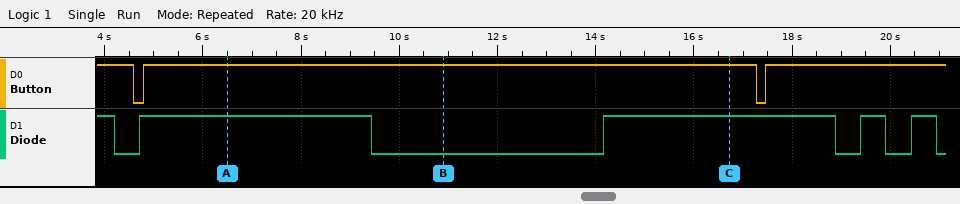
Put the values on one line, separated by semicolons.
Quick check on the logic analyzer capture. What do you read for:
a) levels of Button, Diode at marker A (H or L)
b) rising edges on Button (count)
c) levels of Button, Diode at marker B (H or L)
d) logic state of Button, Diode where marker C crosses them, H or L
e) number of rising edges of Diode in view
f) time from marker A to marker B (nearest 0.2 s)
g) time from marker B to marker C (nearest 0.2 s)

Button=H, Diode=H; 2; Button=H, Diode=L; Button=H, Diode=H; 4; 4.4 s; 5.8 s
